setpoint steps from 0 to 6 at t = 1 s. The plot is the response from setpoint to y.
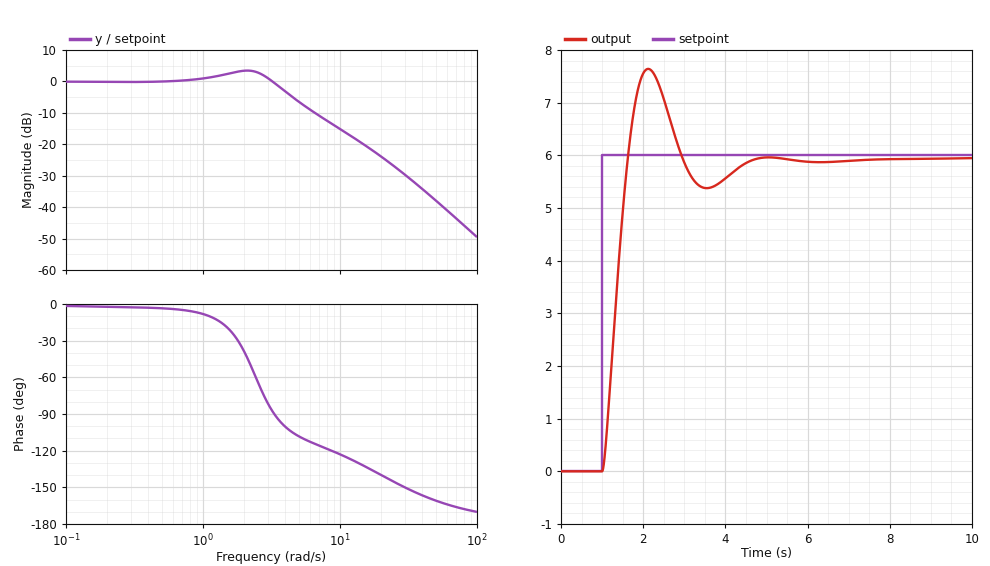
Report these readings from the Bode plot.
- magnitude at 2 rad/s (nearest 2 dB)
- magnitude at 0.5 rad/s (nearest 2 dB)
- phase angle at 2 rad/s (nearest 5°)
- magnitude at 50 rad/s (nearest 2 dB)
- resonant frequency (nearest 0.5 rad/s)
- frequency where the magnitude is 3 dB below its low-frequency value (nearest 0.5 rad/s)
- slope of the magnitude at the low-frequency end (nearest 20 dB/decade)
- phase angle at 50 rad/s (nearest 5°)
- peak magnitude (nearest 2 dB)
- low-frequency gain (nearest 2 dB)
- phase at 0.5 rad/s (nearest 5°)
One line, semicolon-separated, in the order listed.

4 dB; 0 dB; -40°; -38 dB; 2.0 rad/s; 4.0 rad/s; 0 dB/decade; -160°; 4 dB; 0 dB; -5°
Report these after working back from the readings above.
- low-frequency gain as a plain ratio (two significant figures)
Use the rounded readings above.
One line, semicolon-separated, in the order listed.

1.0
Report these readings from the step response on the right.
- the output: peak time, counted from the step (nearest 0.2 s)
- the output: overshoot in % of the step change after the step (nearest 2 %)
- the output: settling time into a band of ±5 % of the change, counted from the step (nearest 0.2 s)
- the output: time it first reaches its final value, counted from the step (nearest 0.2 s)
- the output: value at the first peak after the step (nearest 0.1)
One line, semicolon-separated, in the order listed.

1.2 s; 28 %; 3.2 s; 0.6 s; 7.6
